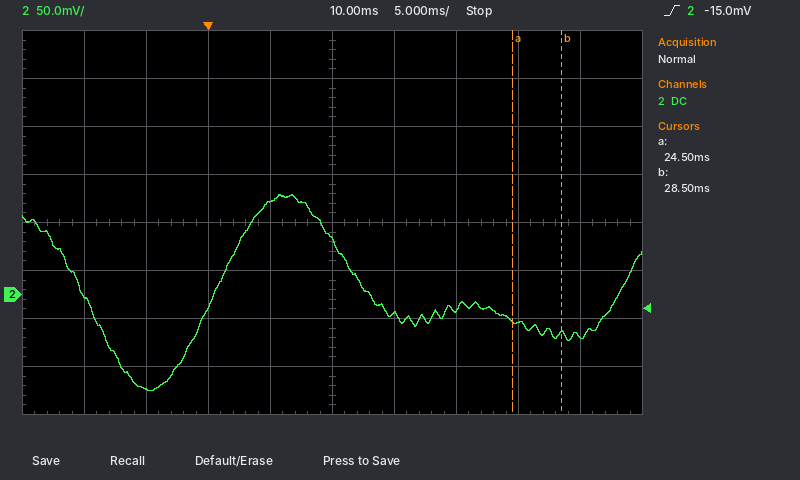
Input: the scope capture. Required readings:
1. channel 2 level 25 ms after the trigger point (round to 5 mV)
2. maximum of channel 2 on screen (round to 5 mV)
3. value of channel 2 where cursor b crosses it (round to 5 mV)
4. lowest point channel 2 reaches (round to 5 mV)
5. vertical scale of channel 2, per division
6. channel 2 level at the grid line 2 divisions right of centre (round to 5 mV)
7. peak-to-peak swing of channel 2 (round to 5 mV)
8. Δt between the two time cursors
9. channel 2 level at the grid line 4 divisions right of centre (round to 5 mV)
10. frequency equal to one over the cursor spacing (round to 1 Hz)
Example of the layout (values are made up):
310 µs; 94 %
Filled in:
-30 mV; 105 mV; -40 mV; -100 mV; 50 mV; -15 mV; 205 mV; 4.0 ms; -45 mV; 250 Hz
